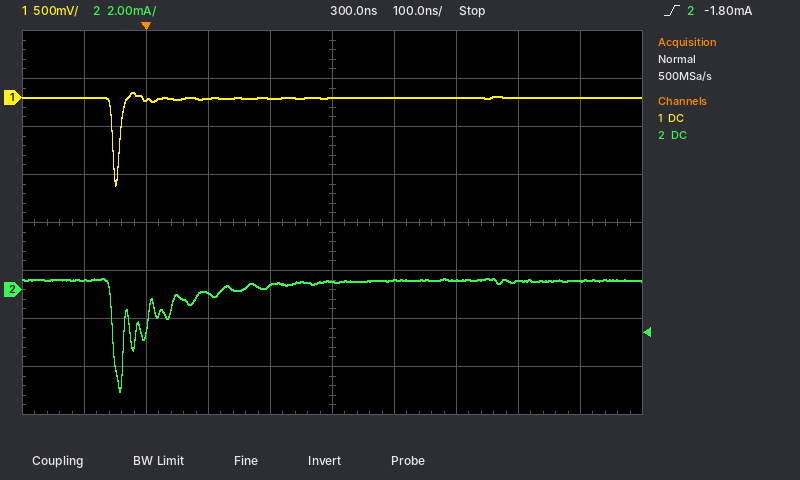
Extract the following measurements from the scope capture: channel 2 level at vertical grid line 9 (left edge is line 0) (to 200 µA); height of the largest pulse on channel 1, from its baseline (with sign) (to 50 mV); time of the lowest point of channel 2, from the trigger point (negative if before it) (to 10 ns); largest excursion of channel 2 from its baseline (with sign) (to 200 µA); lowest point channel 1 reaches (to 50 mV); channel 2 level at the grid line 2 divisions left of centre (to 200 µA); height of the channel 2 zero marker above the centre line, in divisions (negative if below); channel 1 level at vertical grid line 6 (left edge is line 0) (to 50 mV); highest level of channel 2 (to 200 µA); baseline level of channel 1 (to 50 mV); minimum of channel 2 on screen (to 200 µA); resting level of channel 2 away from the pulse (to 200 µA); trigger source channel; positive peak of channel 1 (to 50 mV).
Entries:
400 µA
-900 mV
-40 ns
-4.6 mA
-900 mV
-200 µA
-1.4 div
0 mV
400 µA
0 mV
-4.2 mA
400 µA
channel 2
50 mV
